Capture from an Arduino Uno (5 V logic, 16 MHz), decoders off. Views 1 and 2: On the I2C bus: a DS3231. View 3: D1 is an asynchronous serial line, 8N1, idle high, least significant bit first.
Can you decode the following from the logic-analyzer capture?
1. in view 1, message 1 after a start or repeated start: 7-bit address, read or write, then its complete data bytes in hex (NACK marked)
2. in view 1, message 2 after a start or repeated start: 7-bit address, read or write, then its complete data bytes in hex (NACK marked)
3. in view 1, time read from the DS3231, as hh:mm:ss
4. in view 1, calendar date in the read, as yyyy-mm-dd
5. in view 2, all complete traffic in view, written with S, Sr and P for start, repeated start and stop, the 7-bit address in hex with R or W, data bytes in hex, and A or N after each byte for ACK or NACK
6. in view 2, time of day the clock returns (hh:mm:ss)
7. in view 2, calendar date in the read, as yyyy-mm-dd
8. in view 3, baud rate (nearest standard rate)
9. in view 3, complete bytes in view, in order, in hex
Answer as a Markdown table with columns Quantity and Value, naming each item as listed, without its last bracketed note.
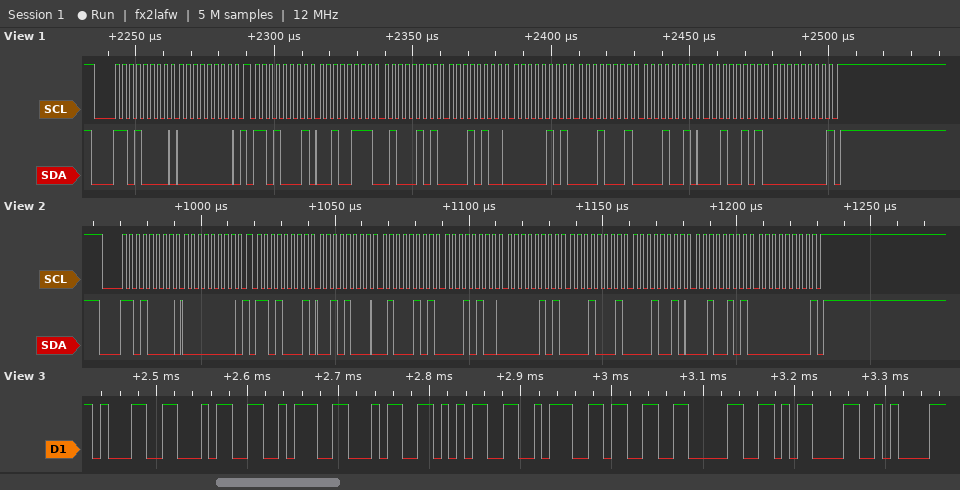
| Quantity | Value |
|---|---|
| in view 1, message 1 after a start or repeated start: 7-bit address, read or write, then its complete data bytes in hex | 0x68 write: 00 |
| in view 1, message 2 after a start or repeated start: 7-bit address, read or write, then its complete data bytes in hex | 0x68 read: 27 45 14 05 11 12 25 00 NACK |
| in view 1, time read from the DS3231, as hh:mm:ss | 14:45:27 |
| in view 1, calendar date in the read, as yyyy-mm-dd | 2025-12-11 |
| in view 2, all complete traffic in view, written with S, Sr and P for start, repeated start and stop, the 7-bit address in hex with R or W, data bytes in hex, and A or N after each byte for ACK or NACK | S 68W A 00 A Sr 68R A 28 A 45 A 14 A 05 A 11 A 12 A 25 A 00 N P |
| in view 2, time of day the clock returns | 14:45:28 |
| in view 2, calendar date in the read, as yyyy-mm-dd | 2025-12-11 |
| in view 3, baud rate | 115200 baud |
| in view 3, complete bytes in view, in order, in hex | 31 34 3A 34 35 3A 33 30 0D 0A |
